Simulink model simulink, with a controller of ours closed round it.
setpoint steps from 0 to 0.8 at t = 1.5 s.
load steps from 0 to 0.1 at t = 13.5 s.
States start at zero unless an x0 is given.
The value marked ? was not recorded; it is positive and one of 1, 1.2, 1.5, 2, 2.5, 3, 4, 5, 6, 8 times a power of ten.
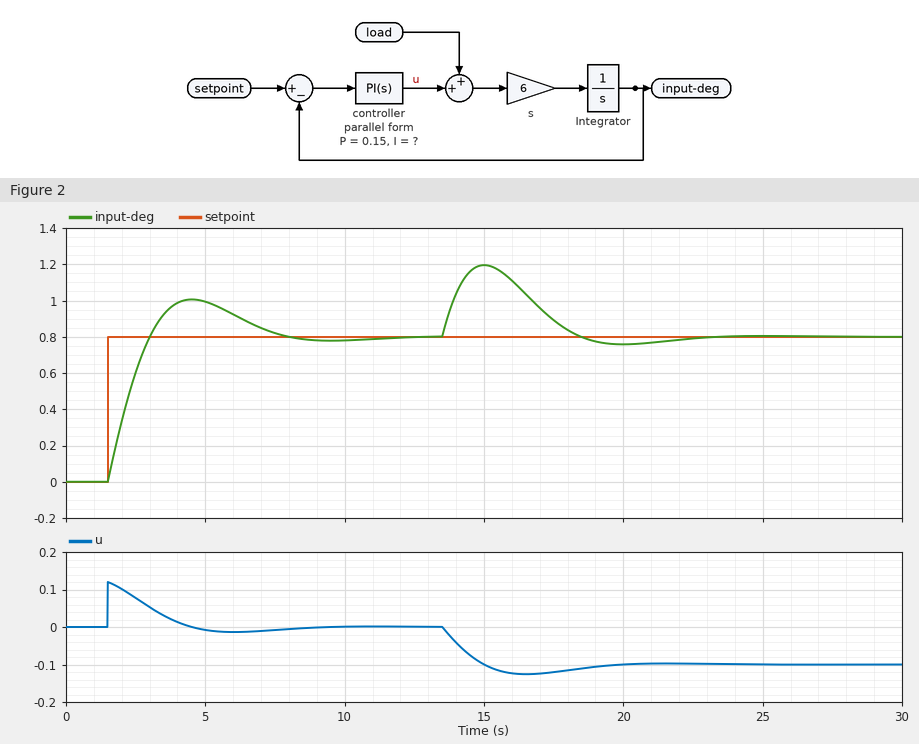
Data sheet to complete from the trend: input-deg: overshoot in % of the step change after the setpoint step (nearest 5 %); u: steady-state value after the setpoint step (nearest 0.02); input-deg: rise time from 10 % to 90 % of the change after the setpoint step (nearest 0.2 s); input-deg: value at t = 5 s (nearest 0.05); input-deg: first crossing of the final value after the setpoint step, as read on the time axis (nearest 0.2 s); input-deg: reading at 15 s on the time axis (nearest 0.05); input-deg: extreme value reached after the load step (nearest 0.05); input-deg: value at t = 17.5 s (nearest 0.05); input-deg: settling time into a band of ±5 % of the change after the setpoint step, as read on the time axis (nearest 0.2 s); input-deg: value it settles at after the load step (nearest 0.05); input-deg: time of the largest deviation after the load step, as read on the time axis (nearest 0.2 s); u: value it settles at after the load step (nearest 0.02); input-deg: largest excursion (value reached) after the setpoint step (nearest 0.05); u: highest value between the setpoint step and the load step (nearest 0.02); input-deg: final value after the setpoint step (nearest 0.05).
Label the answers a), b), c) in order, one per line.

a) 25 %
b) 0.00
c) 1.2 s
d) 1.00
e) 3.0 s
f) 1.20
g) 1.20
h) 0.90
i) 7.2 s
j) 0.80
k) 15.0 s
l) -0.10
m) 1.00
n) 0.12
o) 0.80
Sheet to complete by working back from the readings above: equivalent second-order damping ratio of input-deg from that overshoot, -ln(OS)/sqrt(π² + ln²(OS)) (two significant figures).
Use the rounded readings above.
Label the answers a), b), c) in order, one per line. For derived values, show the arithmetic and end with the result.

a) ln(0.25) = -1.386; 1.386 / sqrt(9.870 + 1.922) = 0.40
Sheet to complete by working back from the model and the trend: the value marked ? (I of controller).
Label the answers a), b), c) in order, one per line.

a) 0.1
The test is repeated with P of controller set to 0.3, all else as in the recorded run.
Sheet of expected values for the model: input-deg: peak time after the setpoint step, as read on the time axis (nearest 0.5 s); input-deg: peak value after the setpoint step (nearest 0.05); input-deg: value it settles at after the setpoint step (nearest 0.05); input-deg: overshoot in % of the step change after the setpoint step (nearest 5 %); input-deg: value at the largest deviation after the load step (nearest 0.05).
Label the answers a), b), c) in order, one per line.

a) 4.0 s
b) 0.90
c) 0.80
d) 10 %
e) 1.05
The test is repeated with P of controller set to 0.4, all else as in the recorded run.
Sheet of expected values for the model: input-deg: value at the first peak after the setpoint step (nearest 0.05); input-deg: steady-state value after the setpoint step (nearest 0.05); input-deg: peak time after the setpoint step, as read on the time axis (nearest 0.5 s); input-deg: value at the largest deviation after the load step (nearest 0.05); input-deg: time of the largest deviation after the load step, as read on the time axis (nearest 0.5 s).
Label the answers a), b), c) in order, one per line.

a) 0.85
b) 0.80
c) 3.5 s
d) 1.00
e) 14.5 s
